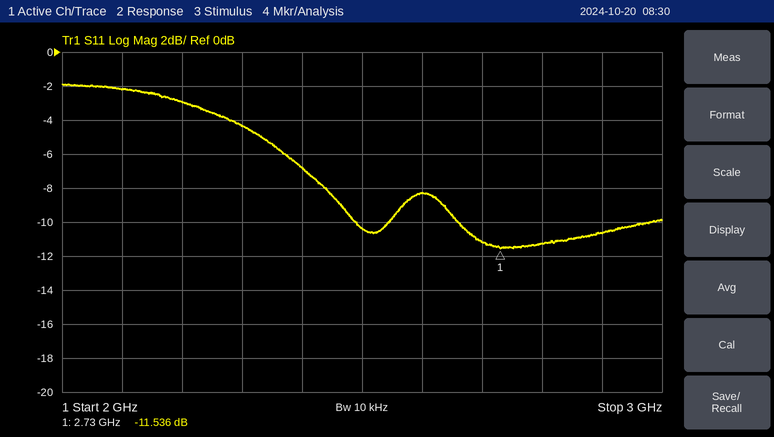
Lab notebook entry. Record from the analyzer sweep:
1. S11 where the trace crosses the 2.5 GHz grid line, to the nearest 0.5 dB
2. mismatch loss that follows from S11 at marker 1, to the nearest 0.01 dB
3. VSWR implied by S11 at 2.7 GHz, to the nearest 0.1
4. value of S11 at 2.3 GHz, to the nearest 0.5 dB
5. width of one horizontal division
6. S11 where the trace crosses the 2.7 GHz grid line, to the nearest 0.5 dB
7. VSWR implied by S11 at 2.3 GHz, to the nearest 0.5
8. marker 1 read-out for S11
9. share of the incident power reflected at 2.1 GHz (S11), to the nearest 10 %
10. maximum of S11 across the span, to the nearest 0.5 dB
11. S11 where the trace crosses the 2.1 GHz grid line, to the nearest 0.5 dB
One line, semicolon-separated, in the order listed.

-10.5 dB; 0.32 dB; 1.8; -4.5 dB; 100 MHz; -11.0 dB; 4.0; -11.536 dB; 60 %; -2.0 dB; -2.0 dB
